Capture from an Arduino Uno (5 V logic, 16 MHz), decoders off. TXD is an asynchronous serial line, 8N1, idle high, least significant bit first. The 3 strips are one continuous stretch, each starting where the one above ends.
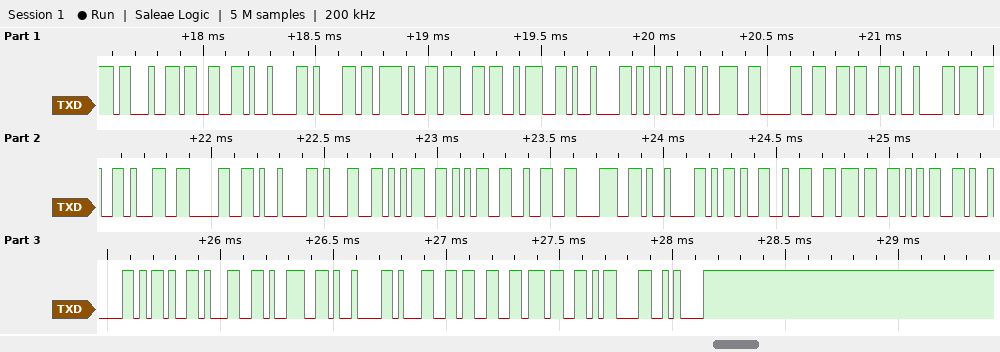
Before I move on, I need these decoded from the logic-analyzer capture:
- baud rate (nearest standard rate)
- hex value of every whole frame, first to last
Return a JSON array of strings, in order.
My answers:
["38400 baud", "23 33 09 61 2F 67 3A 09 2D 39 30 36 09 37 31 30 09 31 35 35 32 38 09 2D 32 37 35 09 2D 31 39 09 31 33 37 0D 0A"]
